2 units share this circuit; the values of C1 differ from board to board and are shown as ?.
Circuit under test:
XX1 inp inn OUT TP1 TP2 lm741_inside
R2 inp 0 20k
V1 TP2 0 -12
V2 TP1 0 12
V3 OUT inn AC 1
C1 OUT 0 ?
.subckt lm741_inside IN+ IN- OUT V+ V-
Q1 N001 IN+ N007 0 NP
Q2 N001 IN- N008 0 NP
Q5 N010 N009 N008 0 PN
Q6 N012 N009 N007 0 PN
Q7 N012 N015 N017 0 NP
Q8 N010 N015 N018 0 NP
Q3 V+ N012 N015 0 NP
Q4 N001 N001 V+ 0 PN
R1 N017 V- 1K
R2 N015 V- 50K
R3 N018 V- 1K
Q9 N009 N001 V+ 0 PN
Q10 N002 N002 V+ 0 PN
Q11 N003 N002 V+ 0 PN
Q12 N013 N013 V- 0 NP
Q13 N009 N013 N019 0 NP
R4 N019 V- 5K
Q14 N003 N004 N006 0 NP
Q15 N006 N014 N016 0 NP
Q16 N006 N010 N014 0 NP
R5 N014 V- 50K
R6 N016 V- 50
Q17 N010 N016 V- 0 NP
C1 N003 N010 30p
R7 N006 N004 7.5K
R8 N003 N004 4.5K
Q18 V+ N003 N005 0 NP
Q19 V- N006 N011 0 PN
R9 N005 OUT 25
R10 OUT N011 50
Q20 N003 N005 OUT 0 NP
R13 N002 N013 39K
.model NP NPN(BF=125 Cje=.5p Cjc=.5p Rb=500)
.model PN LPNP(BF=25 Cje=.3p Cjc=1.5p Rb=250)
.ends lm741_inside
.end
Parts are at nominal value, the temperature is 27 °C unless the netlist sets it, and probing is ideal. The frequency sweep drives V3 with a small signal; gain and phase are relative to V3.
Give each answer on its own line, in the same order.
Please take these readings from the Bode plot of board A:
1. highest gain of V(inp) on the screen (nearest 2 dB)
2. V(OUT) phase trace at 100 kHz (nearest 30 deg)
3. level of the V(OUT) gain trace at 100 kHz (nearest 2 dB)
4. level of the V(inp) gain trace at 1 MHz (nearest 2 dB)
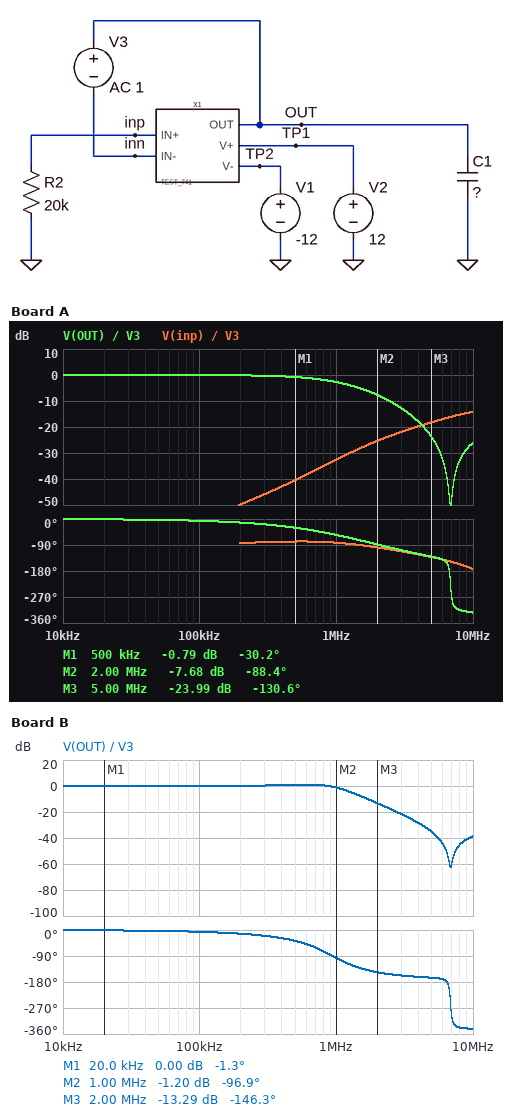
-14 dB
0 deg
0 dB
-32 dB
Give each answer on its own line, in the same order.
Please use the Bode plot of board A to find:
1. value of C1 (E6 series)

3.3 pF
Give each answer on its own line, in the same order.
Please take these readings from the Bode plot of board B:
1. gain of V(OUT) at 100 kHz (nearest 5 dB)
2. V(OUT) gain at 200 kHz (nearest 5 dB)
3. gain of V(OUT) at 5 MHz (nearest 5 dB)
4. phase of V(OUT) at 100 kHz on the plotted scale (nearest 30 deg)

0 dB
0 dB
-35 dB
0 deg
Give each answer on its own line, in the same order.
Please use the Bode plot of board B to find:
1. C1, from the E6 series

22 pF
